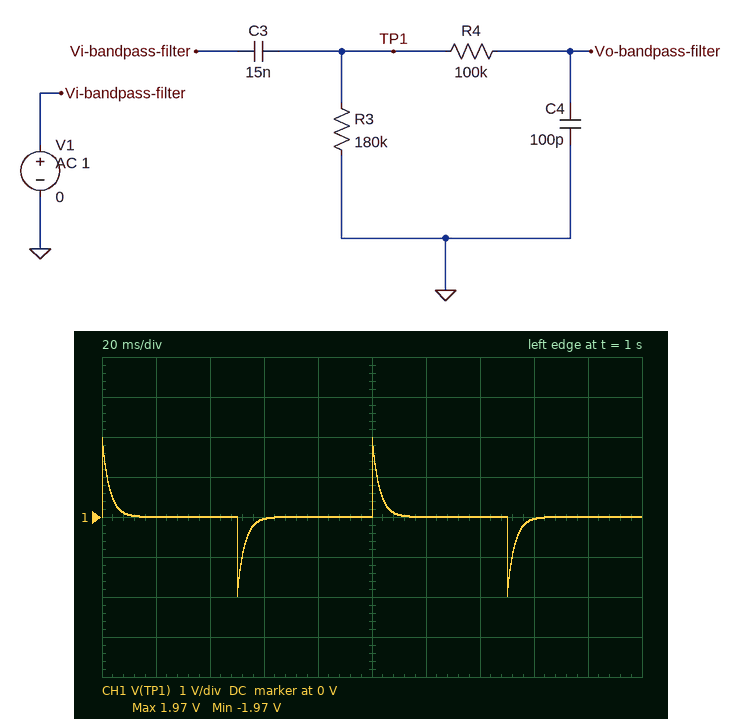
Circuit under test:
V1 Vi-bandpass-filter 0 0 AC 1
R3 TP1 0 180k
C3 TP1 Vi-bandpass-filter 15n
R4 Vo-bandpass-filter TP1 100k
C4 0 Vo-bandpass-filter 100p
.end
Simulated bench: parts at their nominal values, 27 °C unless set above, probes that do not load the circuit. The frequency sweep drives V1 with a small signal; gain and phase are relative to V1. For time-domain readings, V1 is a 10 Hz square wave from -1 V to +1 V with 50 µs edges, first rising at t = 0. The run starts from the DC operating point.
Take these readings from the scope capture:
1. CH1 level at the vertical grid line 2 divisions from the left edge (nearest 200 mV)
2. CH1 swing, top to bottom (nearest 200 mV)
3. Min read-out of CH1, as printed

0 V
4.0 V
-1.97 V
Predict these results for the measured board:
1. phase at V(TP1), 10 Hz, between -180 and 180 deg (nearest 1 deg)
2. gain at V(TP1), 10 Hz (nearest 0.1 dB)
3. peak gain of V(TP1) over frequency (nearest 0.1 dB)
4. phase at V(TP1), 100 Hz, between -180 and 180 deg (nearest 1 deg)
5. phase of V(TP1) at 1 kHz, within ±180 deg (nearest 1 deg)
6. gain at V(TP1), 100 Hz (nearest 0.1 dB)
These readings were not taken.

80 deg
-15.5 dB
0 dB
30 deg
3 deg
-1.3 dB
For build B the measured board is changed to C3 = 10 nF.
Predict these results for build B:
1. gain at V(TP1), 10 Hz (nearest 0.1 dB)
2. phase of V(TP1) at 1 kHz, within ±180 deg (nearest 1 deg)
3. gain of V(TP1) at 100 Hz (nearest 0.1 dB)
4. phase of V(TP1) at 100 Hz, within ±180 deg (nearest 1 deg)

-19.0 dB
5 deg
-2.6 dB
41 deg
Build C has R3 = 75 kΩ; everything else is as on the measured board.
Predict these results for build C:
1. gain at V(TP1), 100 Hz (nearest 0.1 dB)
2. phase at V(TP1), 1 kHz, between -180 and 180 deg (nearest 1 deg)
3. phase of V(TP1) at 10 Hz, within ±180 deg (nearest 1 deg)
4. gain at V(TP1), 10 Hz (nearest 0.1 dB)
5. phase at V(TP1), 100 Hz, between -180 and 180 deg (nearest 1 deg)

-4.8 dB
8 deg
86 deg
-23.0 dB
55 deg
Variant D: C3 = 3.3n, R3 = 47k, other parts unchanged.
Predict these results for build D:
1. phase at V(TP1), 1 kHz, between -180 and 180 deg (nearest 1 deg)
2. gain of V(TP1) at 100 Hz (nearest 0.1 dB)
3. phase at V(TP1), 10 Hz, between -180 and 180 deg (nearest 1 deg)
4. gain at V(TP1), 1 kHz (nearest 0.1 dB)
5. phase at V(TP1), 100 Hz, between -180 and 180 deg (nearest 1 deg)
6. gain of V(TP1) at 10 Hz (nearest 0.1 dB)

45 deg
-20.3 dB
89 deg
-3.3 dB
84 deg
-40.2 dB
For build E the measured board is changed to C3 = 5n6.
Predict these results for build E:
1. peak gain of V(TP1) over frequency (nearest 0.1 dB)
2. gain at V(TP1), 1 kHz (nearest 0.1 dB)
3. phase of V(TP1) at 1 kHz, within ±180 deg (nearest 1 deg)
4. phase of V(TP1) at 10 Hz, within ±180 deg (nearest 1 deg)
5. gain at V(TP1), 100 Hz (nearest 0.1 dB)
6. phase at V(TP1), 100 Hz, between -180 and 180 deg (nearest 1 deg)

0 dB
-0.3 dB
9 deg
86 deg
-5.5 dB
57 deg
